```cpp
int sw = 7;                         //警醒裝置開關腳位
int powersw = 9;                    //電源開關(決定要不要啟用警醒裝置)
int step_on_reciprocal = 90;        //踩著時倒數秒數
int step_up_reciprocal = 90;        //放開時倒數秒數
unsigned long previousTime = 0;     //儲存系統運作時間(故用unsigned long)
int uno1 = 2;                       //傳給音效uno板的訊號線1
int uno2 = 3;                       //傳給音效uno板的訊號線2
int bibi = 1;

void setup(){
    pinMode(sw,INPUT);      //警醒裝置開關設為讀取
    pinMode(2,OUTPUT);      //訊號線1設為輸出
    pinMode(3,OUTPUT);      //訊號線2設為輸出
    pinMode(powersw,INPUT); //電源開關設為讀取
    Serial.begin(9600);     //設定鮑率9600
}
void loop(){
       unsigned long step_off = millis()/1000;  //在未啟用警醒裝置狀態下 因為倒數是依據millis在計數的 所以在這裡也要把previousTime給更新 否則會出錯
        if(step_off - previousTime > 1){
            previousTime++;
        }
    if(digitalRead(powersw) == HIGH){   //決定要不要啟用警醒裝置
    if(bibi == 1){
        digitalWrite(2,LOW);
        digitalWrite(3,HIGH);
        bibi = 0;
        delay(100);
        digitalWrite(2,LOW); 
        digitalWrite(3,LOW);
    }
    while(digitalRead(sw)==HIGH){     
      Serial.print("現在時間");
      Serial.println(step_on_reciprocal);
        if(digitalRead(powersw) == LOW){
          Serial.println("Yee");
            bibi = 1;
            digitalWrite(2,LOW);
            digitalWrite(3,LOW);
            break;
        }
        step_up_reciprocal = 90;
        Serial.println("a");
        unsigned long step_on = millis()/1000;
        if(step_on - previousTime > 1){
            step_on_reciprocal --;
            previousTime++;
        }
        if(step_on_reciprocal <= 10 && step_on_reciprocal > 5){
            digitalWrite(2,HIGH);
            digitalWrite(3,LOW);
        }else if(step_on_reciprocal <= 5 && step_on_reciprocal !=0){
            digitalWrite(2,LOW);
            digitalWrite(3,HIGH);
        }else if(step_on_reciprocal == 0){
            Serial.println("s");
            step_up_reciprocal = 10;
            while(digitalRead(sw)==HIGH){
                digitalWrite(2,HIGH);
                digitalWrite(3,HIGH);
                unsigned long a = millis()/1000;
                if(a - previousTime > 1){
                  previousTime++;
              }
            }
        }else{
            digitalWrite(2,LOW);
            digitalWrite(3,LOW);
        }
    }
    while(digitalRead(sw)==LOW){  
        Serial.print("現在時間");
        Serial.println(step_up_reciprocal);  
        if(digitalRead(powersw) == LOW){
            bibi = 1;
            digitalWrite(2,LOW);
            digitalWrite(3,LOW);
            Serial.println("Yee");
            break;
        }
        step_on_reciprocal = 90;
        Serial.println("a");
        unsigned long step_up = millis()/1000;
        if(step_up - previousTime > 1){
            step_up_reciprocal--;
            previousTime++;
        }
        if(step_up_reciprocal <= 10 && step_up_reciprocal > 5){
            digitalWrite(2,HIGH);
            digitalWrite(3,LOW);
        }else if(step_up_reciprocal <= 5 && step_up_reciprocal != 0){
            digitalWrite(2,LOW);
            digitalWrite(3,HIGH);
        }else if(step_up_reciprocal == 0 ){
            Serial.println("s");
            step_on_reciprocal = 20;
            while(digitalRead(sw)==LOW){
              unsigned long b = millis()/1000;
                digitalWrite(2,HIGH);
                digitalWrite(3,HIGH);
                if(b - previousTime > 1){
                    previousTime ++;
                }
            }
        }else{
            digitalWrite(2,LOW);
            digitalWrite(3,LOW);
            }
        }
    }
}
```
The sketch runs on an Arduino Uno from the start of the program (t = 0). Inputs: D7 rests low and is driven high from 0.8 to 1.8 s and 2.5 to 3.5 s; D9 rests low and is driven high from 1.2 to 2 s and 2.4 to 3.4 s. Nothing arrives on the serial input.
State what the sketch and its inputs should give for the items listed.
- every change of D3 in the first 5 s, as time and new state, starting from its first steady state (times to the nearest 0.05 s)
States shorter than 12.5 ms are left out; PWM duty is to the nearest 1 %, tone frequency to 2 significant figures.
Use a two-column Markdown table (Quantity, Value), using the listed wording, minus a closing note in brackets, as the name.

| Quantity | Value |
|---|---|
| every change of D3 in the first 5 s, as time and new state, starting from its first steady state | 0 s low; 1.2 s high; 1.3 s low; 2.4 s high; 2.5 s low |
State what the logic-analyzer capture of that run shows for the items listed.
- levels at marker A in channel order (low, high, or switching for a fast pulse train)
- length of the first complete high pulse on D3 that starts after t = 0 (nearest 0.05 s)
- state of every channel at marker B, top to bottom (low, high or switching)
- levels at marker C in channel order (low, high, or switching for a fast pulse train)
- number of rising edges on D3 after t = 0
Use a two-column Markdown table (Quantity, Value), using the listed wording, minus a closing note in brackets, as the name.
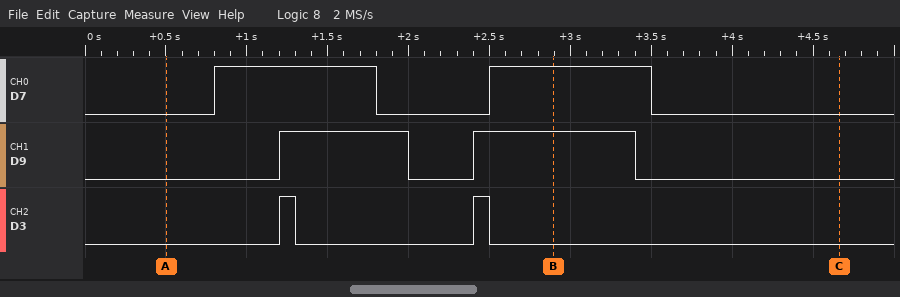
| Quantity | Value |
|---|---|
| levels at marker A in channel order | D7 low, D9 low, D3 low |
| length of the first complete high pulse on D3 that starts after t = 0 | 0.10 s |
| state of every channel at marker B, top to bottom | D7 high, D9 high, D3 low |
| levels at marker C in channel order | D7 low, D9 low, D3 low |
| number of rising edges on D3 after t = 0 | 2 |
